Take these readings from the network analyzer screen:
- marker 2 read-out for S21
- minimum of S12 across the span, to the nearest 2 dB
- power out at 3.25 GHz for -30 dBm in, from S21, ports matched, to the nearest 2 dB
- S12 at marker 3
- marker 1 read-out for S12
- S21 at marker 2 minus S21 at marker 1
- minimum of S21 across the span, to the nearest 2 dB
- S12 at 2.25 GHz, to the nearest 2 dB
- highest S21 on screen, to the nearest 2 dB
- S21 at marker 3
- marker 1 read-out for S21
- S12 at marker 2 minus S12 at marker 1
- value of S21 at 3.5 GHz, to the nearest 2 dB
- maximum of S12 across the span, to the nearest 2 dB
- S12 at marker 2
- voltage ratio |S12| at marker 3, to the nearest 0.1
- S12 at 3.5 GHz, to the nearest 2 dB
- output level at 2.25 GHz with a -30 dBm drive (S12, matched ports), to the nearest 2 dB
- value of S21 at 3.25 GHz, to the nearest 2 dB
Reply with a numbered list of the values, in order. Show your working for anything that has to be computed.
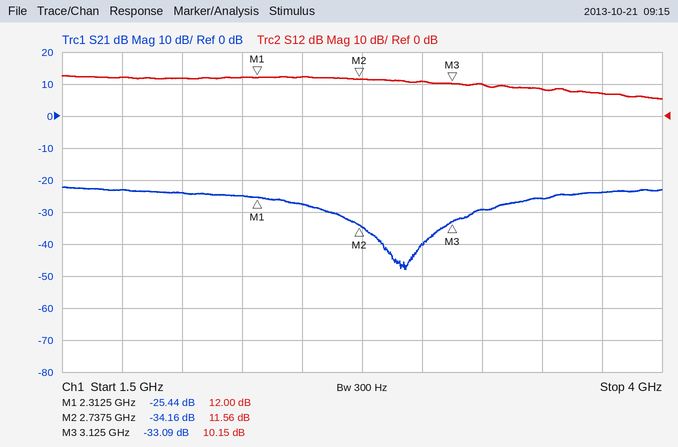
1. -34.16 dB
2. 6 dB
3. -30 dBm + (-30 dB) = -60 dBm
4. 10.15 dB
5. 12.00 dB
6. -34.16 − (-25.44) = -8.72 dB
7. -48 dB
8. 12 dB
9. -22 dB
10. -33.09 dB
11. -25.44 dB
12. 11.56 − (12) = -0.44 dB
13. -26 dB
14. 12 dB
15. 11.56 dB
16. 10^(10.15/20) ≈ 3.2
17. 8 dB
18. -30 dBm + (12 dB) = -18 dBm
19. -30 dB
